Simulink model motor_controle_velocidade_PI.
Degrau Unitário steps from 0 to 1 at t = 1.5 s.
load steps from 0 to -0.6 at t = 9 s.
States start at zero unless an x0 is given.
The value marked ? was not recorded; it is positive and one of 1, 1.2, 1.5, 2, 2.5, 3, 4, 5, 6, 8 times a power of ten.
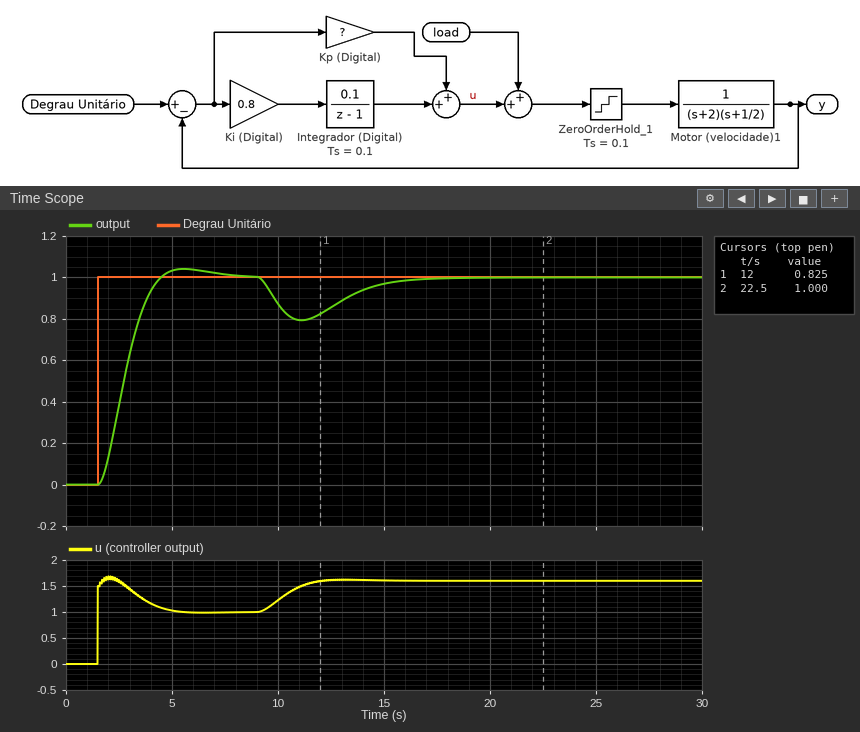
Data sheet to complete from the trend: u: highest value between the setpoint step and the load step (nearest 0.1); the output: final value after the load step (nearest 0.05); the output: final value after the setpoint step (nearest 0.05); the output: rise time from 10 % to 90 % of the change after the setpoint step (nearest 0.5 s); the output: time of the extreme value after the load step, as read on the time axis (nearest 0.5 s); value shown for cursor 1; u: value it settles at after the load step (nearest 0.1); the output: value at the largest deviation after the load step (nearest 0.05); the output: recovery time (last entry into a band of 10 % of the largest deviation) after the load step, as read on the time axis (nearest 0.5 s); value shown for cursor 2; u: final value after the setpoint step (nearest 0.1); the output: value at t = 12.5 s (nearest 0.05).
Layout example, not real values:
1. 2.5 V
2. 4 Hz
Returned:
1. 1.7
2. 1.00
3. 1.00
4. 2.0 s
5. 11.0 s
6. 0.825
7. 1.6
8. 0.80
9. 15.5 s
10. 1.000
11. 1.0
12. 0.85
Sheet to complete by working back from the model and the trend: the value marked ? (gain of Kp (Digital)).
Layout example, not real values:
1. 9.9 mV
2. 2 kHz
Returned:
1. 1.5
